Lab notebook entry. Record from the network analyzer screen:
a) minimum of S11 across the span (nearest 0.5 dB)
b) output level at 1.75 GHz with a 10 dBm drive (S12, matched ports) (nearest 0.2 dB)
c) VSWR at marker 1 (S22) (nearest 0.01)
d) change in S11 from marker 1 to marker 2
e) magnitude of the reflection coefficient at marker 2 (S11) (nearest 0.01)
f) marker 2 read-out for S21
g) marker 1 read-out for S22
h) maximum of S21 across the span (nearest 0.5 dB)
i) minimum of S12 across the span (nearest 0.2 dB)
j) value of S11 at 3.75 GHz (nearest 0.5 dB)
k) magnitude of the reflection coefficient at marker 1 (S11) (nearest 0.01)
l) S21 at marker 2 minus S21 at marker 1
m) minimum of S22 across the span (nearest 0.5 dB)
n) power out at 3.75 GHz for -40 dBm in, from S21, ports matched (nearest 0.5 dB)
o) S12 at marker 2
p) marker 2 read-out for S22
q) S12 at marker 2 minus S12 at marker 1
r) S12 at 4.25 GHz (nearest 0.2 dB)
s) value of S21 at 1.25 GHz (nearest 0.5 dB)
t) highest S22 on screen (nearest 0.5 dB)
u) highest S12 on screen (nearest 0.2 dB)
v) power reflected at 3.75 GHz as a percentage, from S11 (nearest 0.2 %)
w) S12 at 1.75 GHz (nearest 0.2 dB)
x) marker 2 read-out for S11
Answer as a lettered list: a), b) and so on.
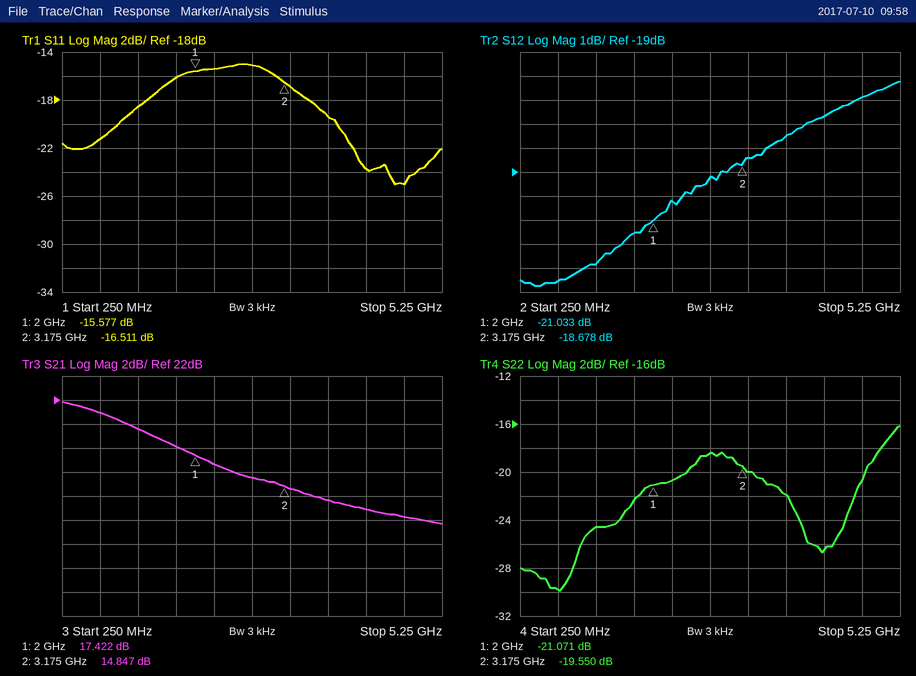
a) -25.0 dB
b) -11.6 dBm
c) 1.19
d) -0.934 dB
e) 0.15
f) 14.847 dB
g) -21.071 dB
h) 22.0 dB
i) -23.8 dB
j) -19.5 dB
k) 0.17
l) -2.575 dB
m) -30.0 dB
n) -26.5 dBm
o) -18.678 dB
p) -19.550 dB
q) 2.355 dB
r) -16.6 dB
s) 19.5 dB
t) -16.0 dB
u) -15.2 dB
v) 1.2 %
w) -21.6 dB
x) -16.511 dB
